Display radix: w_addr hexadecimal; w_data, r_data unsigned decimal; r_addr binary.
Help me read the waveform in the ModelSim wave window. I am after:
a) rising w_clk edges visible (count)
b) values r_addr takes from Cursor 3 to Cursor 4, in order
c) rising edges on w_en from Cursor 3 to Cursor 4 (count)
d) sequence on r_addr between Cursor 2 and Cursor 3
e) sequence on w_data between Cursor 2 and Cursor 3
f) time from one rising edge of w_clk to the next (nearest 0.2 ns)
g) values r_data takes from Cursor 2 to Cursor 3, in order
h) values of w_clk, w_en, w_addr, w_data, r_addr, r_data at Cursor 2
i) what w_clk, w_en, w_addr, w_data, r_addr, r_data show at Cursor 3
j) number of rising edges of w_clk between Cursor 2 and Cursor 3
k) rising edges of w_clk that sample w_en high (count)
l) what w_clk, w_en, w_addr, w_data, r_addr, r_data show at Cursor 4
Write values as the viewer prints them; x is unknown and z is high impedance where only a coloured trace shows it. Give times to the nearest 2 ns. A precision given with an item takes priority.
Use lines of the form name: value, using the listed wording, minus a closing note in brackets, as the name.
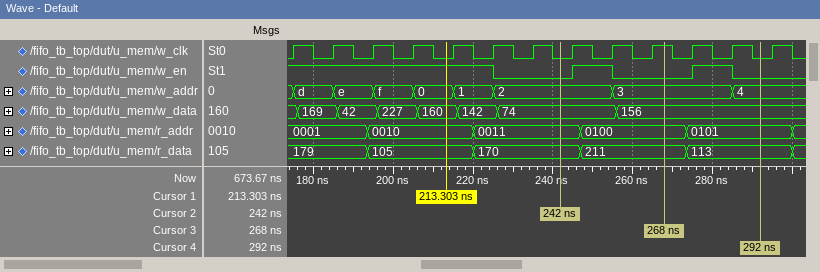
rising w_clk edges visible: 13
values r_addr takes from Cursor 3 to Cursor 4, in order: 0100, 0101
rising edges on w_en from Cursor 3 to Cursor 4: 1
sequence on r_addr between Cursor 2 and Cursor 3: 0011, 0100
sequence on w_data between Cursor 2 and Cursor 3: 74, 156
time from one rising edge of w_clk to the next: 10 ns
values r_data takes from Cursor 2 to Cursor 3, in order: 170, 211
values of w_clk, w_en, w_addr, w_data, r_addr, r_data at Cursor 2: w_clk=0, w_en=0, w_addr=2, w_data=74, r_addr=0011, r_data=170
what w_clk, w_en, w_addr, w_data, r_addr, r_data show at Cursor 3: w_clk=1, w_en=0, w_addr=3, w_data=156, r_addr=0100, r_data=211
number of rising edges of w_clk between Cursor 2 and Cursor 3: 3
rising edges of w_clk that sample w_en high: 8
what w_clk, w_en, w_addr, w_data, r_addr, r_data show at Cursor 4: w_clk=0, w_en=0, w_addr=4, w_data=156, r_addr=0101, r_data=113
